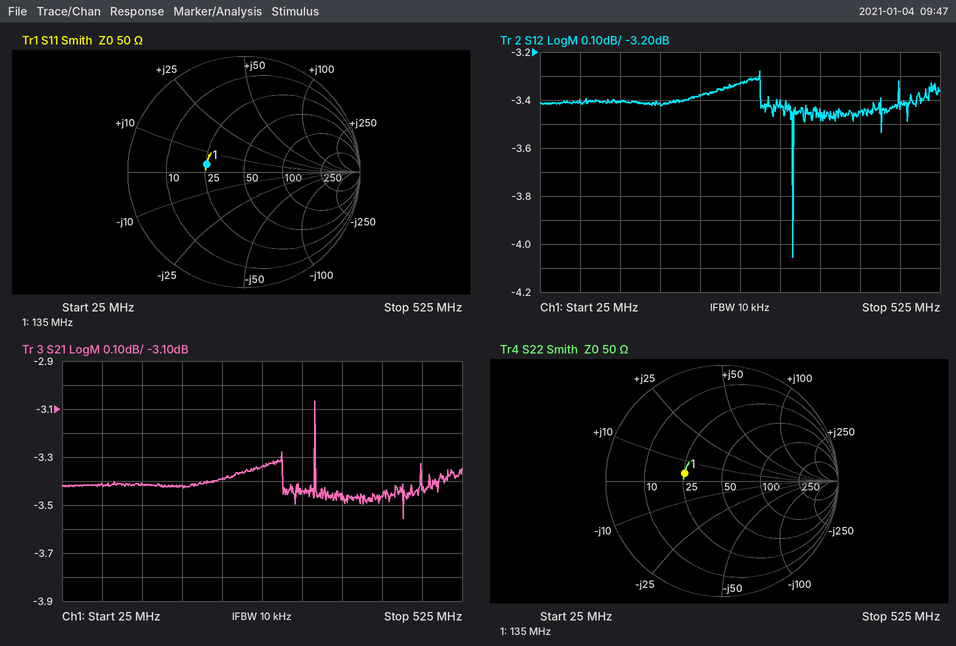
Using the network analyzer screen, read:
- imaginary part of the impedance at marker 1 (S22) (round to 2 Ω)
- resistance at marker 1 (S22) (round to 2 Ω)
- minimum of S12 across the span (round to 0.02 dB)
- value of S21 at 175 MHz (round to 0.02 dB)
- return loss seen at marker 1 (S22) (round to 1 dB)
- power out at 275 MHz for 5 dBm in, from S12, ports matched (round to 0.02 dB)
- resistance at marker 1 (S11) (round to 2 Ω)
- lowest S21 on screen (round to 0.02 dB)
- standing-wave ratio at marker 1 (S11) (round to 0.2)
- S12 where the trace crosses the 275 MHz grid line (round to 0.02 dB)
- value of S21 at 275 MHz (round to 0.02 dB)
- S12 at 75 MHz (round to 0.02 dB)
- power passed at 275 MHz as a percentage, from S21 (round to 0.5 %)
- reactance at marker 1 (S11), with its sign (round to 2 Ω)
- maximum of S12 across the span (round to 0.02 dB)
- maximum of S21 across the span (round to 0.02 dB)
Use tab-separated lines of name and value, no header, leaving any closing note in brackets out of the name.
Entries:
imaginary part of the impedance at marker 1 (S22)	+4 Ω
resistance at marker 1 (S22)	26 Ω
minimum of S12 across the span	-4.06 dB
value of S21 at 175 MHz	-3.42 dB
return loss seen at marker 1 (S22)	10 dB
power out at 275 MHz for 5 dBm in, from S12, ports matched	1.68 dBm
resistance at marker 1 (S11)	26 Ω
lowest S21 on screen	-3.56 dB
standing-wave ratio at marker 1 (S11)	2.0
S12 where the trace crosses the 275 MHz grid line	-3.32 dB
value of S21 at 275 MHz	-3.34 dB
S12 at 75 MHz	-3.40 dB
power passed at 275 MHz as a percentage, from S21	46.5 %
reactance at marker 1 (S11), with its sign	+4 Ω
maximum of S12 across the span	-3.28 dB
maximum of S21 across the span	-3.06 dB
